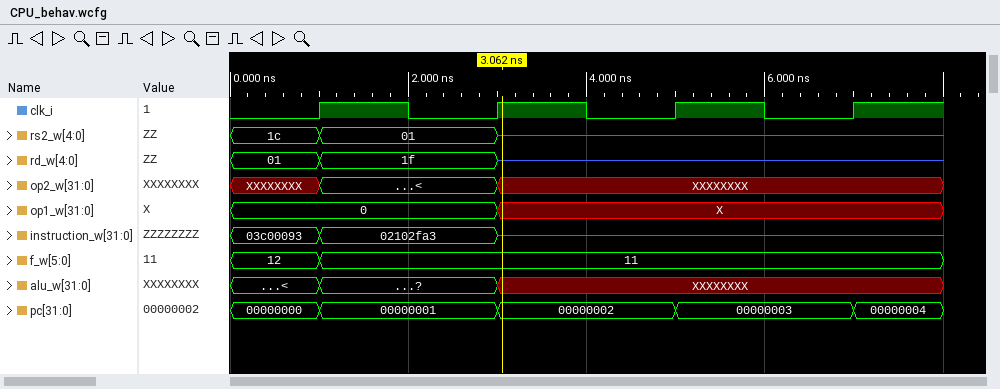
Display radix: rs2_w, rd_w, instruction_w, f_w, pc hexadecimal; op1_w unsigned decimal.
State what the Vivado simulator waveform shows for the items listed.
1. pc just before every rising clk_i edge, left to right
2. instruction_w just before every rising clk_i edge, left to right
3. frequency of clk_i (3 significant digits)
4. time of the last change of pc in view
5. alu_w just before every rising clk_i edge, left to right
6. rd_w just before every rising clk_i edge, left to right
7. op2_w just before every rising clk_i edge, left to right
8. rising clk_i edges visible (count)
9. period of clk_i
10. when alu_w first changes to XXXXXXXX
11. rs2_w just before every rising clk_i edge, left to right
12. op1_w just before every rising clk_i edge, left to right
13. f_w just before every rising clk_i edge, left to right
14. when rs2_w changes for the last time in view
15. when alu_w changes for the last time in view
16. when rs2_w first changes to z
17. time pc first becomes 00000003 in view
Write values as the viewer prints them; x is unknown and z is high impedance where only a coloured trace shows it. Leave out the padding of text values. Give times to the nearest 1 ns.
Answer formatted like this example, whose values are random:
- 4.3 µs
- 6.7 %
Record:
- 00000000, 00000001, 00000002, 00000003
- 03c00093, 02102fa3, z, z
- 500 MHz
- 7 ns
- <, ?, XXXXXXXX, XXXXXXXX
- 01, 1f, z, z
- XXXXXXXX, <, XXXXXXXX, XXXXXXXX
- 4
- 2 ns
- 3 ns
- 1c, 01, z, z
- 0, 0, X, X
- 12, 11, 11, 11
- 3 ns
- 3 ns
- 3 ns
- 5 ns
